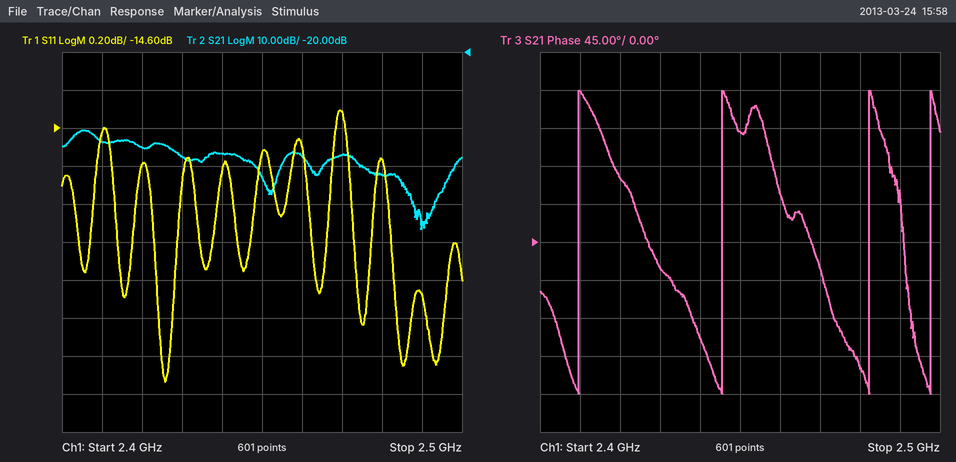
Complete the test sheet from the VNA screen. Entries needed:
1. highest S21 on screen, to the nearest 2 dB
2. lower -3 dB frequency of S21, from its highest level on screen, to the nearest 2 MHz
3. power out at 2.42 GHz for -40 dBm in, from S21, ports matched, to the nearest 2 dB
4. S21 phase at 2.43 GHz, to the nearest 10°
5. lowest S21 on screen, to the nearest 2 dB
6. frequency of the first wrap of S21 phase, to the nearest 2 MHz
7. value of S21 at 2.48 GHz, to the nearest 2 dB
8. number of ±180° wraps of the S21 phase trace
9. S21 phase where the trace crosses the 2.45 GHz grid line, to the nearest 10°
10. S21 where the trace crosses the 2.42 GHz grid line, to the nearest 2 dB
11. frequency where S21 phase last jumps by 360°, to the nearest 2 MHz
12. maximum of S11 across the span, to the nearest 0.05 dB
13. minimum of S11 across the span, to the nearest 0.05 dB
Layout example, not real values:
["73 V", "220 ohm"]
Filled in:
["-40 dB", "2.402 GHz", "-86 dBm", "-30°", "-66 dB", "2.410 GHz", "-52 dB", "4", "130°", "-46 dB", "2.498 GHz", "-14.50 dB", "-15.95 dB"]
